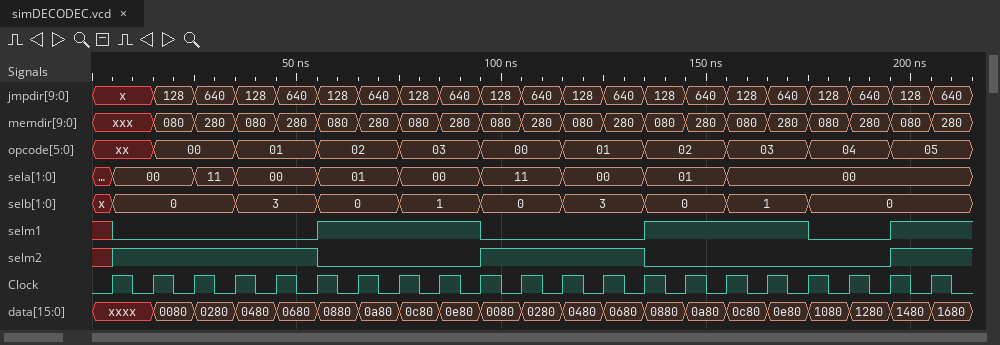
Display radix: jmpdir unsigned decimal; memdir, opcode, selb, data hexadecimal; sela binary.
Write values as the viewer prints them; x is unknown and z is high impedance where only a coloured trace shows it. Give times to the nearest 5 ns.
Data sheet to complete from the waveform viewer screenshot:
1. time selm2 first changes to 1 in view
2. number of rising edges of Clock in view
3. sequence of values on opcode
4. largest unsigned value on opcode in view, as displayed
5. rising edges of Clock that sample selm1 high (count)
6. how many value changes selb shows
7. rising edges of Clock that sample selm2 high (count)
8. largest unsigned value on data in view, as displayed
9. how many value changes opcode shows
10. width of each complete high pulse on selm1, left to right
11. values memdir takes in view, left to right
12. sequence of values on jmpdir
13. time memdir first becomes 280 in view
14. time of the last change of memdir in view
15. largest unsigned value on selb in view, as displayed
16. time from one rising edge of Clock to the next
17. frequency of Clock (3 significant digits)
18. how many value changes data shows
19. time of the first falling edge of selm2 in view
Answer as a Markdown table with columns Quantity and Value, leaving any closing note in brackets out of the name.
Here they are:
| Quantity | Value |
|---|---|
| time selm2 first changes to 1 in view | 5 ns |
| number of rising edges of Clock in view | 21 |
| sequence of values on opcode | xx, 00, 01, 02, 03, 00, 01, 02, 03, 04, 05 |
| largest unsigned value on opcode in view, as displayed | 05 |
| rising edges of Clock that sample selm1 high | 9 |
| how many value changes selb shows | 9 |
| rising edges of Clock that sample selm2 high | 10 |
| largest unsigned value on data in view, as displayed | 1680 |
| how many value changes opcode shows | 10 |
| width of each complete high pulse on selm1, left to right | 40 ns, 40 ns |
| values memdir takes in view, left to right | xxx, 080, 280, 080, 280, 080, 280, 080, 280, 080, 280, 080, 280, 080, 280, 080, 280, 080, 280, 080, 280 |
| sequence of values on jmpdir | x, 128, 640, 128, 640, 128, 640, 128, 640, 128, 640, 128, 640, 128, 640, 128, 640, 128, 640, 128, 640 |
| time memdir first becomes 280 in view | 25 ns |
| time of the last change of memdir in view | 205 ns |
| largest unsigned value on selb in view, as displayed | 3 |
| time from one rising edge of Clock to the next | 10 ns |
| frequency of Clock | 100 MHz |
| how many value changes data shows | 20 |
| time of the first falling edge of selm2 in view | 55 ns |
